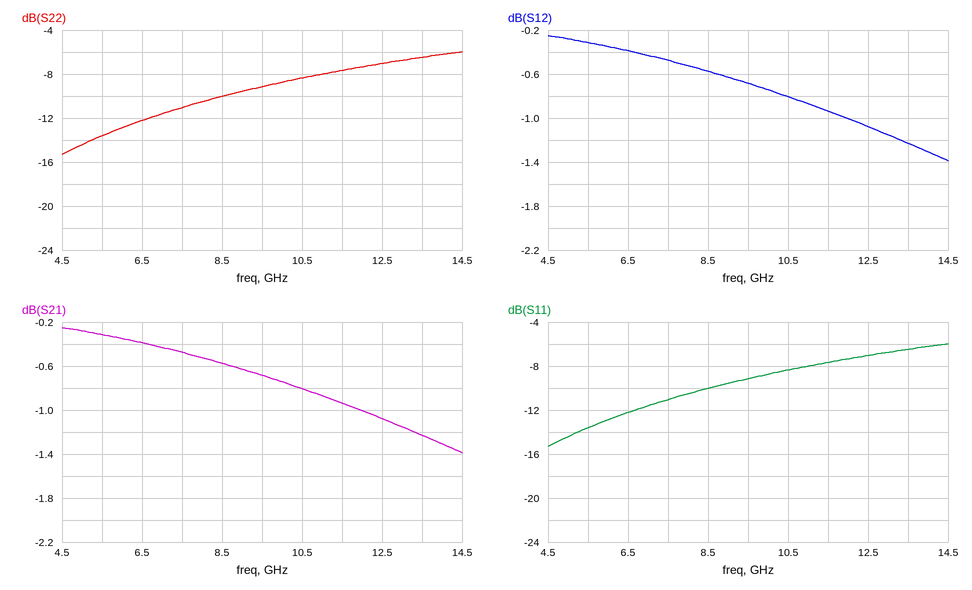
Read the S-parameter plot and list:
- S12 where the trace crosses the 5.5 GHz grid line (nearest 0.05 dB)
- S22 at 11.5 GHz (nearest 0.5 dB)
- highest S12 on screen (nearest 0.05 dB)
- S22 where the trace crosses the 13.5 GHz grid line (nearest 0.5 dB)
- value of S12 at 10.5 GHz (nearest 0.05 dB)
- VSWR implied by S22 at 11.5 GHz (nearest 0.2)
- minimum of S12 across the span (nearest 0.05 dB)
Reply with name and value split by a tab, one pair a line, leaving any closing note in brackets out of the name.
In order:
S12 where the trace crosses the 5.5 GHz grid line	-0.30 dB
S22 at 11.5 GHz	-7.5 dB
highest S12 on screen	-0.25 dB
S22 where the trace crosses the 13.5 GHz grid line	-6.5 dB
value of S12 at 10.5 GHz	-0.80 dB
VSWR implied by S22 at 11.5 GHz	2.4
minimum of S12 across the span	-1.40 dB
